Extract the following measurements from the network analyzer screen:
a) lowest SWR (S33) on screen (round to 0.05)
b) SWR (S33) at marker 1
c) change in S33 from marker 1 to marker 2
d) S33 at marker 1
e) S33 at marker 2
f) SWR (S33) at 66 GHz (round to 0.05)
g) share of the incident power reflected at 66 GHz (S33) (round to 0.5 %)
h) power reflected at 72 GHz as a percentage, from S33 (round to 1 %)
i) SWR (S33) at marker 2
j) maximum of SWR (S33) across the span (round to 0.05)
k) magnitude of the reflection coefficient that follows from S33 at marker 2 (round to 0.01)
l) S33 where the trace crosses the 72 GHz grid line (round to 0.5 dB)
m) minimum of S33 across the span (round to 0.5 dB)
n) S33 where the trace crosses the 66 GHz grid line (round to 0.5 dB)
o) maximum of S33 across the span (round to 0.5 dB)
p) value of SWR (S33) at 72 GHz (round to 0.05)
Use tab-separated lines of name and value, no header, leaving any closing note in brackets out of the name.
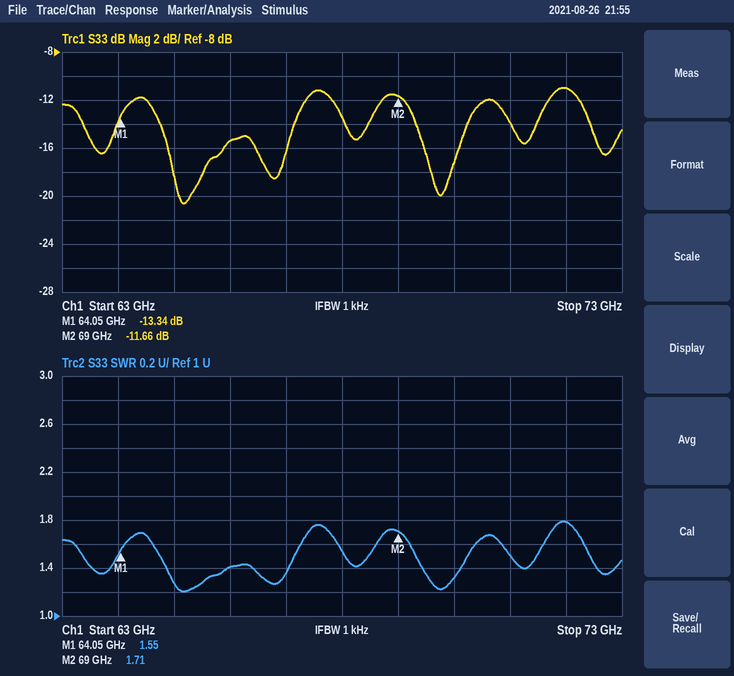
lowest SWR (S33) on screen	1.20
SWR (S33) at marker 1	1.55
change in S33 from marker 1 to marker 2	1.68 dB
S33 at marker 1	-13.34 dB
S33 at marker 2	-11.66 dB
SWR (S33) at 66 GHz	1.40
share of the incident power reflected at 66 GHz (S33)	3.0 %
power reflected at 72 GHz as a percentage, from S33	8 %
SWR (S33) at marker 2	1.71
maximum of SWR (S33) across the span	1.80
magnitude of the reflection coefficient that follows from S33 at marker 2	0.26
S33 where the trace crosses the 72 GHz grid line	-11.0 dB
minimum of S33 across the span	-20.5 dB
S33 where the trace crosses the 66 GHz grid line	-15.5 dB
maximum of S33 across the span	-11.0 dB
value of SWR (S33) at 72 GHz	1.80
